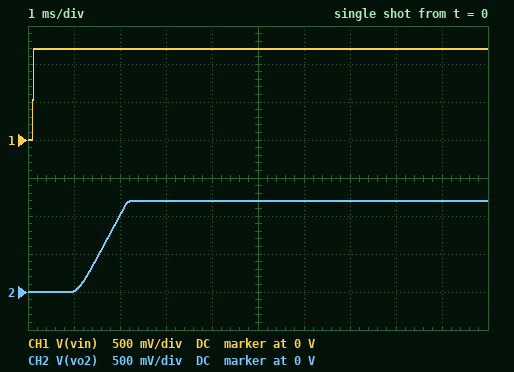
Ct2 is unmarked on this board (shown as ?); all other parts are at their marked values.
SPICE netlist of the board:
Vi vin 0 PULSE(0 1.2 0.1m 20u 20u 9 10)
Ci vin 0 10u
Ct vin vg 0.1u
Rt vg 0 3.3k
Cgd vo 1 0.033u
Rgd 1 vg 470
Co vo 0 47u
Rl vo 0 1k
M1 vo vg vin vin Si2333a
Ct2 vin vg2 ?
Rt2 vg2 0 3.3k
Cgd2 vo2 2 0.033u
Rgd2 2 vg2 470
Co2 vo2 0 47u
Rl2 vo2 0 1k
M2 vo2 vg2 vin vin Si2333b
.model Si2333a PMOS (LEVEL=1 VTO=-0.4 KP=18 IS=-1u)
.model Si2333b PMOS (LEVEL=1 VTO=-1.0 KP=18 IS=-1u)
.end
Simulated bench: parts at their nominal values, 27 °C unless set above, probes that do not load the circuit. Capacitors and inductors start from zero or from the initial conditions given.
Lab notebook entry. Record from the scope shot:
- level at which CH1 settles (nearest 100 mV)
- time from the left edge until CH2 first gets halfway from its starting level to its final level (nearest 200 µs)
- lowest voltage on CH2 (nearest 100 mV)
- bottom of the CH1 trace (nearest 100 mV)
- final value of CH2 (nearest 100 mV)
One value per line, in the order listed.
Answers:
1.2 V
1.6 ms
0 V
0 V
1.2 V
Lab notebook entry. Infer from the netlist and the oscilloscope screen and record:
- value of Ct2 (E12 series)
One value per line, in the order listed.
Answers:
120 nF
